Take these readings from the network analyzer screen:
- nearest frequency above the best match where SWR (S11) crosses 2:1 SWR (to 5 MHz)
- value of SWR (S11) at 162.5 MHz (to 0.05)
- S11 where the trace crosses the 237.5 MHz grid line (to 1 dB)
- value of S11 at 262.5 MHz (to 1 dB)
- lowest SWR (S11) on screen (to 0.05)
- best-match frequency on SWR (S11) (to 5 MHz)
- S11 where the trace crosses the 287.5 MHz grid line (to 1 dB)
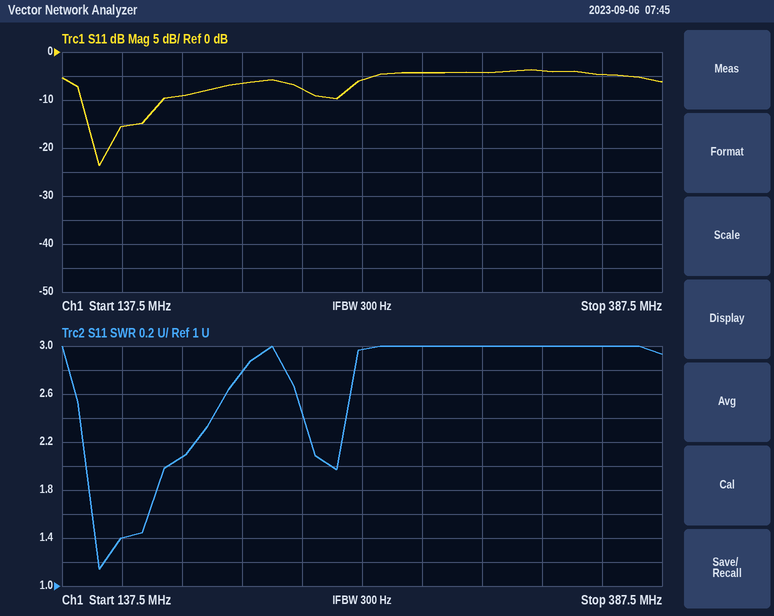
180 MHz
1.40
-8 dB
-6 dB
1.15
155 MHz
-4 dB
